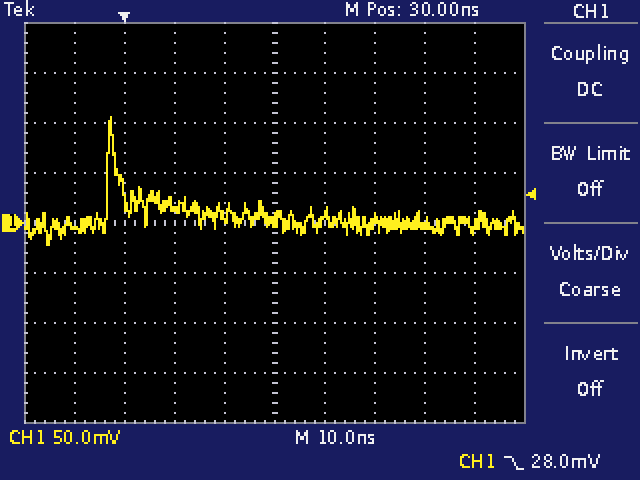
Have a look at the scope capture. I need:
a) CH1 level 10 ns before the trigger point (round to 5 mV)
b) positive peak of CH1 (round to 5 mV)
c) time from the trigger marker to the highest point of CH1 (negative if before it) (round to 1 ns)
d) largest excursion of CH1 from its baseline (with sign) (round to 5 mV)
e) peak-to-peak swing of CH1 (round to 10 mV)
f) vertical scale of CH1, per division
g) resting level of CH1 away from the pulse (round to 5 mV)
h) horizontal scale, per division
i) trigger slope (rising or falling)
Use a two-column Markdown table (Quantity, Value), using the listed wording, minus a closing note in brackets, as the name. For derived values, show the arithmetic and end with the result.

| Quantity | Value |
|---|---|
| CH1 level 10 ns before the trigger point | -5 mV |
| positive peak of CH1 | 105 mV |
| time from the trigger marker to the highest point of CH1 (negative if before it) | -3 ns |
| largest excursion of CH1 from its baseline (with sign) | 105 mV − (0 mV) = +105 mV |
| peak-to-peak swing of CH1 | 130 mV |
| vertical scale of CH1, per division | 50 mV |
| resting level of CH1 away from the pulse | 0 mV |
| horizontal scale, per division | 10 ns |
| trigger slope | falling |
